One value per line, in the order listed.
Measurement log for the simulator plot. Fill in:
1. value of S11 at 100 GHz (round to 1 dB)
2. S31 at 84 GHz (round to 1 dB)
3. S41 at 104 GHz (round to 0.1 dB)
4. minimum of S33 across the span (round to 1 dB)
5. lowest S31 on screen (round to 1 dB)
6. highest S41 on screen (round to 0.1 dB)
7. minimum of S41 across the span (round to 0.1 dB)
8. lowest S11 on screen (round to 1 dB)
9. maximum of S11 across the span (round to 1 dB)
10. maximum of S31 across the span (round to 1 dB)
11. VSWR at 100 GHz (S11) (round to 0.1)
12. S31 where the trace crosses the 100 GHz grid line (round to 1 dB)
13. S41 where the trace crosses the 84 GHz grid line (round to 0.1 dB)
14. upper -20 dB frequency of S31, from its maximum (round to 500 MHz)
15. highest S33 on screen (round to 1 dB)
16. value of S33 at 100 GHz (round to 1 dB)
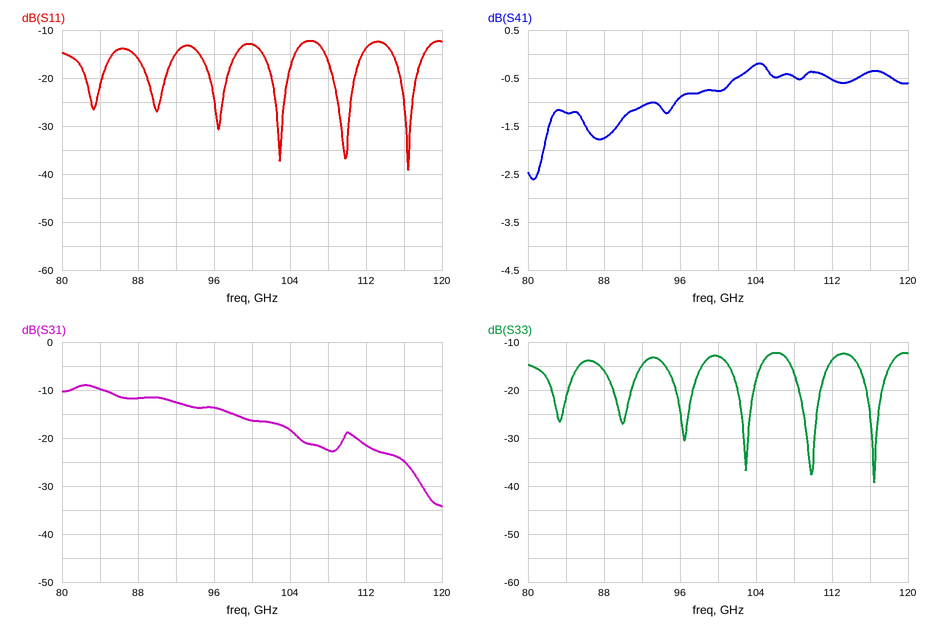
-13 dB
-10 dB
-0.2 dB
-39 dB
-34 dB
-0.2 dB
-2.6 dB
-39 dB
-12 dB
-9 dB
1.6
-16 dB
-1.2 dB
117.5 GHz
-12 dB
-13 dB
